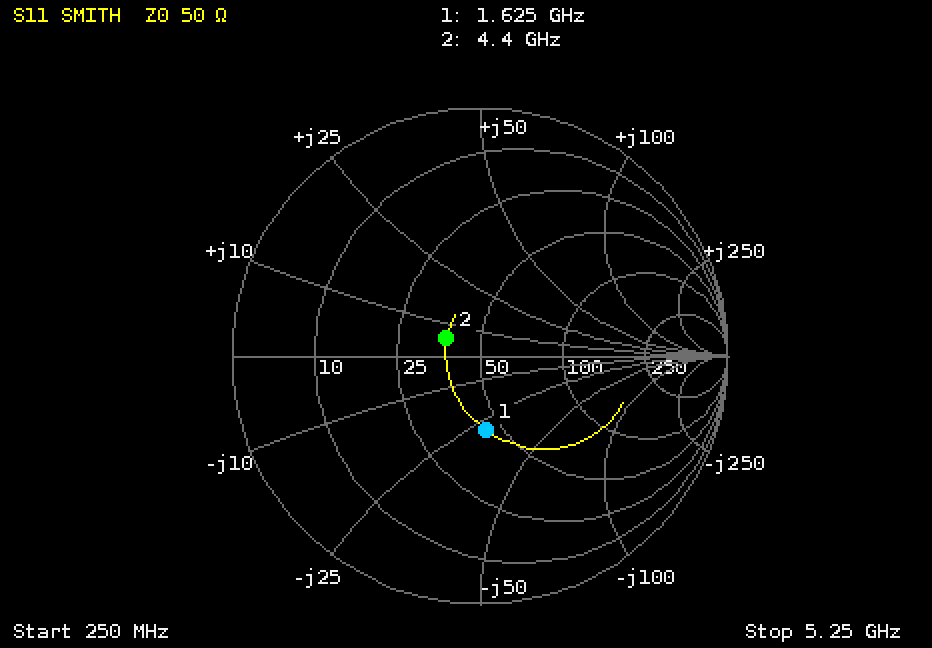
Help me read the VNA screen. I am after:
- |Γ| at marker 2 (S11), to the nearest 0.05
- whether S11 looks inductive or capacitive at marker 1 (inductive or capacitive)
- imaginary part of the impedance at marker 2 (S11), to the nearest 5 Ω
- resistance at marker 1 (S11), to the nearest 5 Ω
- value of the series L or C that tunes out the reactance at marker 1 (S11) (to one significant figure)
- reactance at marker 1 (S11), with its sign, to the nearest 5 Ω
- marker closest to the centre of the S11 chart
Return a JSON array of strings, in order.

["0.15", "capacitive", "+5 Ω", "45 Ω", "3 nH", "-30 Ω", "marker 2"]
